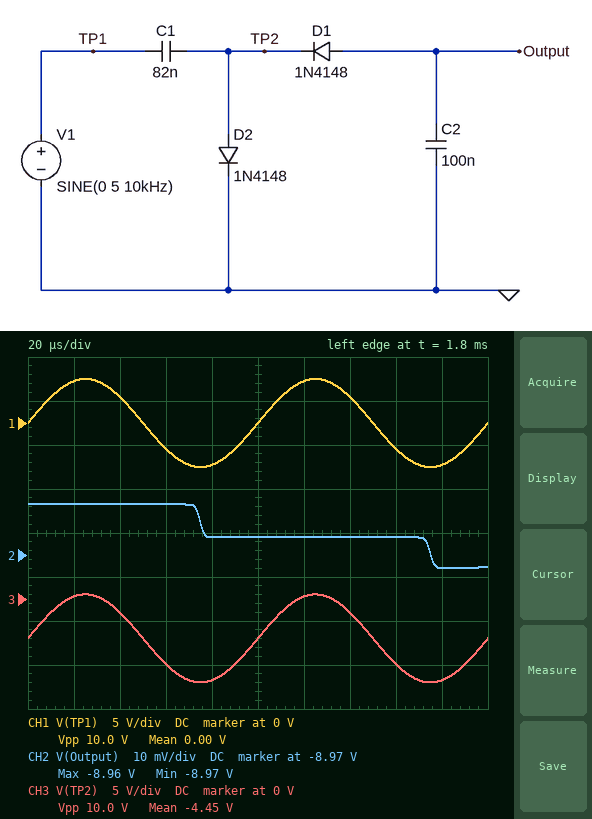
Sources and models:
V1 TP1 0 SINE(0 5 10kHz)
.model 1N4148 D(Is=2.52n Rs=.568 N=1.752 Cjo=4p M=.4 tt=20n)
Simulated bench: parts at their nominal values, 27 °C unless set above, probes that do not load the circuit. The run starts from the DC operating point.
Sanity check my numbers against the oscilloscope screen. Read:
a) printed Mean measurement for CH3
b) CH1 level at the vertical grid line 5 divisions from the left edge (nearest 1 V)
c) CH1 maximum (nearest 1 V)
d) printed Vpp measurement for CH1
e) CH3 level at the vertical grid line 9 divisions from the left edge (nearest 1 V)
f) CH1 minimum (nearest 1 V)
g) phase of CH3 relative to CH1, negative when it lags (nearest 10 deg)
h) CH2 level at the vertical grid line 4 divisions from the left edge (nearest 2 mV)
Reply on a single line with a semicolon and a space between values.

-4.45 V; 0 V; 5 V; 10.0 V; -9 V; -5 V; 0 deg; -8.966 V
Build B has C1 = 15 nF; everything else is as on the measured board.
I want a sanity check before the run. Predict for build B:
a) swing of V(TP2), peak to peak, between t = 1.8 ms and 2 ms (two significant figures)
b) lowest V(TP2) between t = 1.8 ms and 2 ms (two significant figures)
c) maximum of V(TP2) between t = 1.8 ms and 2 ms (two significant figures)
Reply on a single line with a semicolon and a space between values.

9.6 V; -9.0 V; 620 mV
